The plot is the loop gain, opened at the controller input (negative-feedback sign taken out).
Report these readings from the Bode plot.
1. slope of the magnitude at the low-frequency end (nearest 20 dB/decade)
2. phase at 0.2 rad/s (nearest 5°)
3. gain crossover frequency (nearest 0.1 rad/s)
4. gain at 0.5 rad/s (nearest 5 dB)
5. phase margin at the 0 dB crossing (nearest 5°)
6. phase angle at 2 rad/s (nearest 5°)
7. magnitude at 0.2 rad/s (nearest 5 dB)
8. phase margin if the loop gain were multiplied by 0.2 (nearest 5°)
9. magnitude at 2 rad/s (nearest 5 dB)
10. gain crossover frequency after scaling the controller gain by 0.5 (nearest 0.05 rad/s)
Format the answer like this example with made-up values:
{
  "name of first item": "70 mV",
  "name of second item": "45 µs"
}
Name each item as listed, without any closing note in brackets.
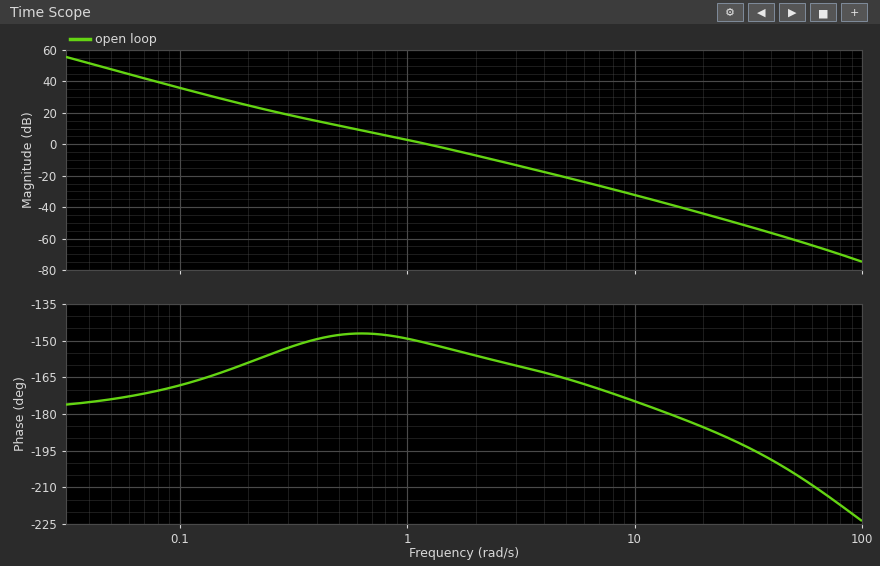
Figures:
{
  "slope of the magnitude at the low-frequency end": "-40 dB/decade",
  "phase at 0.2 rad/s": "-160°",
  "gain crossover frequency": "1.2 rad/s",
  "gain at 0.5 rad/s": "10 dB",
  "phase margin at the 0 dB crossing": "30°",
  "phase angle at 2 rad/s": "-155°",
  "magnitude at 0.2 rad/s": "25 dB",
  "phase margin if the loop gain were multiplied by 0.2": "30°",
  "magnitude at 2 rad/s": "-5 dB",
  "gain crossover frequency after scaling the controller gain by 0.5": "0.80 rad/s"
}
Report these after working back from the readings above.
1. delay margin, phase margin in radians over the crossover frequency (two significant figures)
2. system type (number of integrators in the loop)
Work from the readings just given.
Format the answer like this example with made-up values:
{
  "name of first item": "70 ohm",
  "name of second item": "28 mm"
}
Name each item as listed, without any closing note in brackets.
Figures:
{
  "delay margin, phase margin in radians over the crossover frequency": "0.44 s",
  "system type": "2"
}
